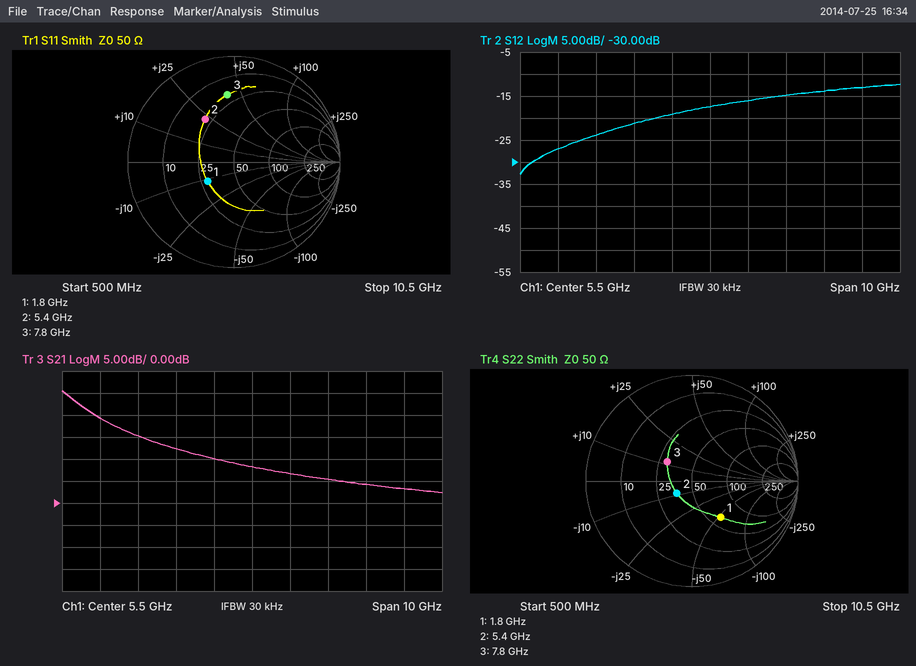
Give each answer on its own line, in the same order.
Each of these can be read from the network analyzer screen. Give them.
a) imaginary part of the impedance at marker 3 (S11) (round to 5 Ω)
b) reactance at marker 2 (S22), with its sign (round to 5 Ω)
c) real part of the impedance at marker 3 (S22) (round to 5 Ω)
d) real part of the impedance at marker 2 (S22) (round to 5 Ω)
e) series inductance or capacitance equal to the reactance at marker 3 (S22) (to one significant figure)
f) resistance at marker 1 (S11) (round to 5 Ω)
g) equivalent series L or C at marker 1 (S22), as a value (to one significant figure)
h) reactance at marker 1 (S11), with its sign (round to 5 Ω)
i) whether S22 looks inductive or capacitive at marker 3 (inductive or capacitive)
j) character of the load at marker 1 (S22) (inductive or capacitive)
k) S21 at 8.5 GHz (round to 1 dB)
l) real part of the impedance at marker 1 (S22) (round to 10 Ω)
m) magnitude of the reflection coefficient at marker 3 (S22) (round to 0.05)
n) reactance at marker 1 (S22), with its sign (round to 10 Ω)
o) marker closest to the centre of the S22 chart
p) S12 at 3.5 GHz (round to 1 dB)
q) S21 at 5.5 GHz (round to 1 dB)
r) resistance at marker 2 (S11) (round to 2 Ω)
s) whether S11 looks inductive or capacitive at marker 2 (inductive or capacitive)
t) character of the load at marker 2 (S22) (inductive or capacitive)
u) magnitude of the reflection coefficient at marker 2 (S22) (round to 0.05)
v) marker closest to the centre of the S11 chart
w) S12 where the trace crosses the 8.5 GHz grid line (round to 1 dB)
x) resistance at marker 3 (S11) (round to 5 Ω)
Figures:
+40 Ω
-10 Ω
30 Ω
35 Ω
200 pH
30 Ω
2 pF
-10 Ω
inductive
capacitive
4 dB
60 Ω
0.30
-50 Ω
marker 2
-21 dB
8 dB
22 Ω
inductive
capacitive
0.20
marker 1
-14 dB
20 Ω
